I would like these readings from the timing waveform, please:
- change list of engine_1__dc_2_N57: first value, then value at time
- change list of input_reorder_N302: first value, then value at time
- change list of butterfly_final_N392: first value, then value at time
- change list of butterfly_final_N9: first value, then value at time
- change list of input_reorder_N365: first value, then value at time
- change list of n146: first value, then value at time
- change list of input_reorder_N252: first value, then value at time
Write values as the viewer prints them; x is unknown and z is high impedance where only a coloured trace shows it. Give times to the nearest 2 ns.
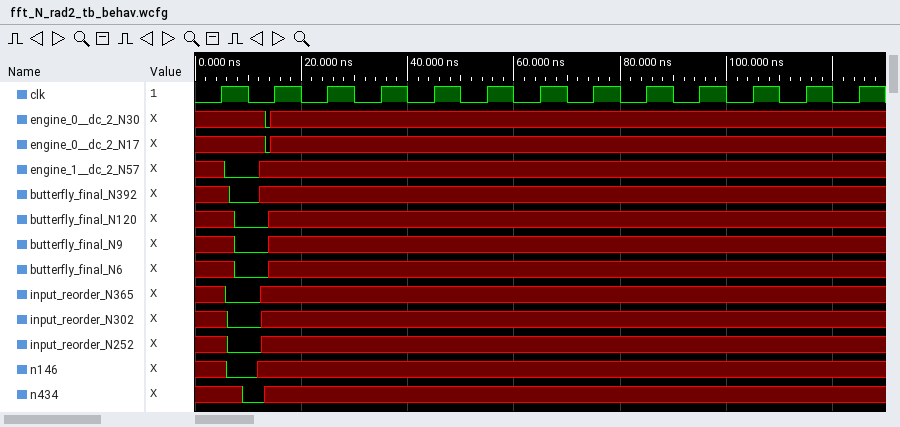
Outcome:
x, 0 at 6 ns, x at 12 ns
x, 0 at 6 ns, x at 12 ns
x, 0 at 6 ns, x at 12 ns
x, 0 at 8 ns, x at 14 ns
x, 0 at 6 ns, x at 12 ns
x, 0 at 6 ns, x at 12 ns
x, 0 at 6 ns, x at 12 ns
